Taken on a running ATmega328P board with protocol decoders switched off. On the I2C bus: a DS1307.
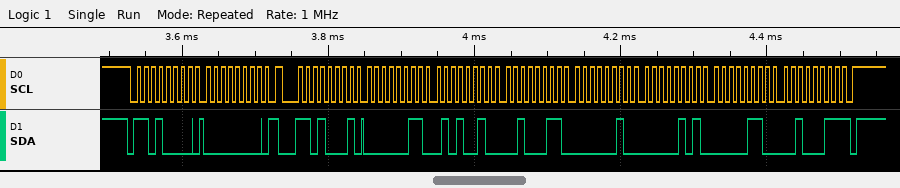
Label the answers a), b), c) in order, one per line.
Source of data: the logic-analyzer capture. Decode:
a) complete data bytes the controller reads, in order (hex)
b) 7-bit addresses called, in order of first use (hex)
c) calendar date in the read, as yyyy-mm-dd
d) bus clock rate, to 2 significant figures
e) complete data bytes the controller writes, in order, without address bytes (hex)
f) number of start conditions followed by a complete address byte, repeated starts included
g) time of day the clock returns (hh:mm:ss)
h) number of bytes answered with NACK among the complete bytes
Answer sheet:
a) 03 52 23 02 05 06 23
b) 0x68
c) 2023-06-05
d) 100 kHz
e) 00
f) 2
g) 23:52:03
h) 1
